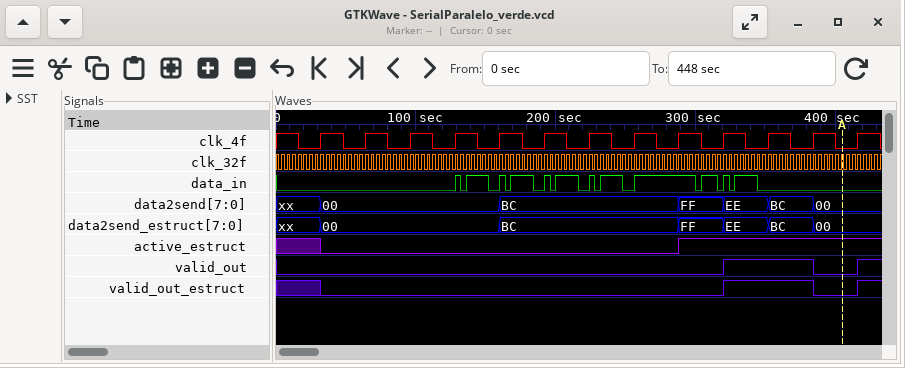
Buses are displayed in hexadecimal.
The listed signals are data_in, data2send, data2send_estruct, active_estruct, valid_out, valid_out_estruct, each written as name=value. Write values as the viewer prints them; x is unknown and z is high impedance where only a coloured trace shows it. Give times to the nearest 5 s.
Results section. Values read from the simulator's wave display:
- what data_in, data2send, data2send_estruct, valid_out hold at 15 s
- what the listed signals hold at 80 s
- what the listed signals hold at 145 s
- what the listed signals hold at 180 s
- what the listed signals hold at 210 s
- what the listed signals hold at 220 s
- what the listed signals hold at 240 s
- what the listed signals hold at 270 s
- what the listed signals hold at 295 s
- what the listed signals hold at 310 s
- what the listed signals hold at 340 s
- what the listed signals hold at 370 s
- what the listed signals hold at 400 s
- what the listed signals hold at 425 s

data_in=0, data2send=xx, data2send_estruct=xx, valid_out=0
data_in=0, data2send=00, data2send_estruct=00, active_estruct=0, valid_out=0, valid_out_estruct=0
data_in=1, data2send=00, data2send_estruct=00, active_estruct=0, valid_out=0, valid_out_estruct=0
data_in=1, data2send=BC, data2send_estruct=BC, active_estruct=0, valid_out=0, valid_out_estruct=0
data_in=1, data2send=BC, data2send_estruct=BC, active_estruct=0, valid_out=0, valid_out_estruct=0
data_in=0, data2send=BC, data2send_estruct=BC, active_estruct=0, valid_out=0, valid_out_estruct=0
data_in=1, data2send=BC, data2send_estruct=BC, active_estruct=0, valid_out=0, valid_out_estruct=0
data_in=1, data2send=BC, data2send_estruct=BC, active_estruct=0, valid_out=0, valid_out_estruct=0
data_in=1, data2send=FF, data2send_estruct=FF, active_estruct=1, valid_out=0, valid_out_estruct=0
data_in=1, data2send=FF, data2send_estruct=FF, active_estruct=1, valid_out=0, valid_out_estruct=0
data_in=1, data2send=EE, data2send_estruct=EE, active_estruct=1, valid_out=1, valid_out_estruct=1
data_in=0, data2send=BC, data2send_estruct=BC, active_estruct=1, valid_out=1, valid_out_estruct=1
data_in=0, data2send=00, data2send_estruct=00, active_estruct=1, valid_out=0, valid_out_estruct=0
data_in=0, data2send=00, data2send_estruct=00, active_estruct=1, valid_out=1, valid_out_estruct=1
